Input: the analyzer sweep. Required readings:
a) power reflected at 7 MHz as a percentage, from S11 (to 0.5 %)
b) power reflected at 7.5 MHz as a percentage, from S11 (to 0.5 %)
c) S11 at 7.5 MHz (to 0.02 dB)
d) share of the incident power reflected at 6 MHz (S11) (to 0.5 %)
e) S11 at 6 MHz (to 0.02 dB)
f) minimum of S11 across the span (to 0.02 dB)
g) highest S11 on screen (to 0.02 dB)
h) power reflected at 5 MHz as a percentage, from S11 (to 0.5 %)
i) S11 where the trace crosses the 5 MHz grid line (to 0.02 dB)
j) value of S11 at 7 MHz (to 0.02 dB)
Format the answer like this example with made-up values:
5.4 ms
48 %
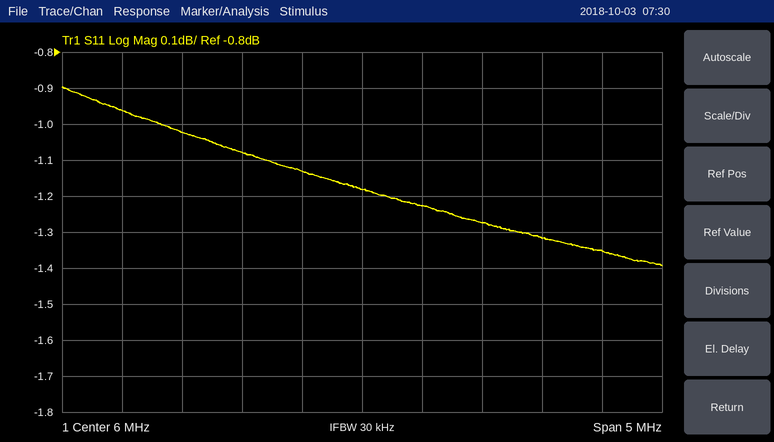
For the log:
74.5 %
74.0 %
-1.32 dB
76.0 %
-1.18 dB
-1.40 dB
-0.90 dB
78.0 %
-1.08 dB
-1.28 dB
